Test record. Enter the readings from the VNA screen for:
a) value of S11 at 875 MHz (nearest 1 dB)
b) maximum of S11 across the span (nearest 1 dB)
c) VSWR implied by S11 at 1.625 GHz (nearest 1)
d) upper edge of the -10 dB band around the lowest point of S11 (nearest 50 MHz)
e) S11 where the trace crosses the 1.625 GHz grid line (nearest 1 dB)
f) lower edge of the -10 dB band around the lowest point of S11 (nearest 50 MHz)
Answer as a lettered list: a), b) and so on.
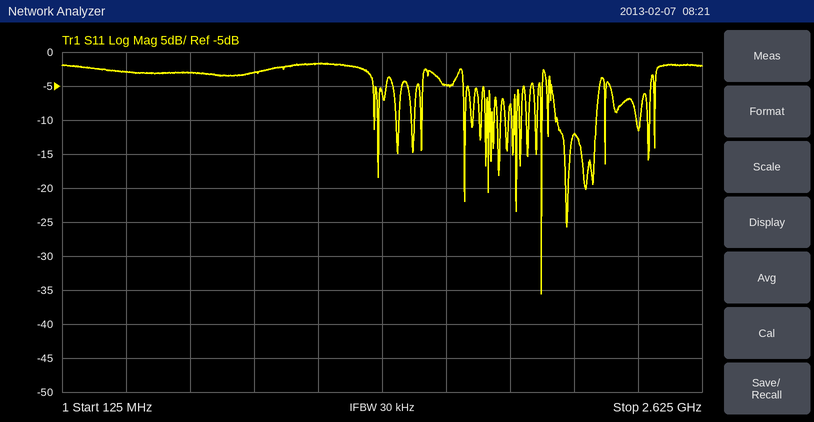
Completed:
a) -3 dB
b) -2 dB
c) 4
d) 2.00 GHz
e) -5 dB
f) 2.00 GHz
